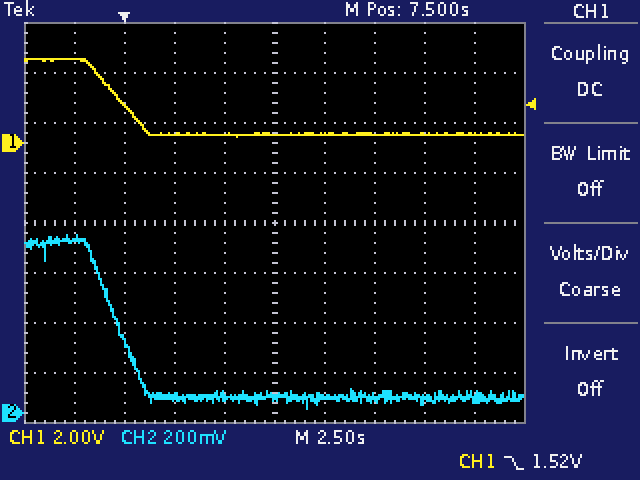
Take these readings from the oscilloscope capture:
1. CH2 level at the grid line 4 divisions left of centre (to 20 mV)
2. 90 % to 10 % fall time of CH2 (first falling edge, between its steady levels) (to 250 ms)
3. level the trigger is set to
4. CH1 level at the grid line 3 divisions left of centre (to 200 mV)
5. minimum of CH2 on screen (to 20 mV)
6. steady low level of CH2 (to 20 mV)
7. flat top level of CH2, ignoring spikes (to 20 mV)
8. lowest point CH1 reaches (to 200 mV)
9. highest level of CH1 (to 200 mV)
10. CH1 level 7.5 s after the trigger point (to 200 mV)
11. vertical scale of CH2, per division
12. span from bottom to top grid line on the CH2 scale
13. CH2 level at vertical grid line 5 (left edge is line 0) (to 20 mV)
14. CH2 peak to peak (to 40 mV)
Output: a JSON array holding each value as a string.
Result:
["700 mV", "2.50 s", "1.52 V", "1.6 V", "20 mV", "60 mV", "680 mV", "200 mV", "3.4 V", "400 mV", "200 mV", "1.6 V", "60 mV", "680 mV"]
